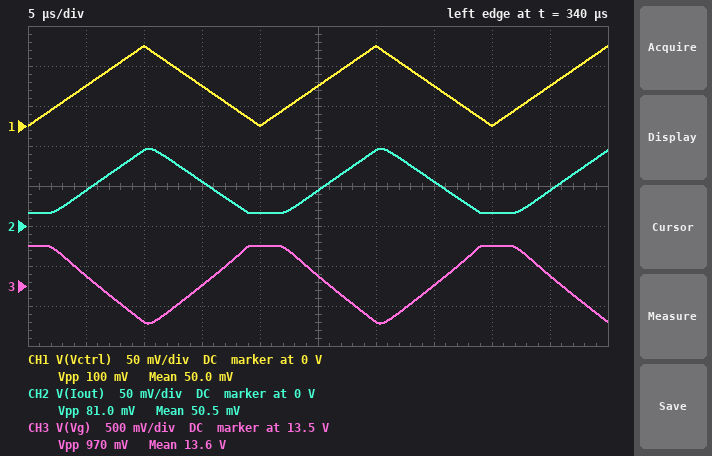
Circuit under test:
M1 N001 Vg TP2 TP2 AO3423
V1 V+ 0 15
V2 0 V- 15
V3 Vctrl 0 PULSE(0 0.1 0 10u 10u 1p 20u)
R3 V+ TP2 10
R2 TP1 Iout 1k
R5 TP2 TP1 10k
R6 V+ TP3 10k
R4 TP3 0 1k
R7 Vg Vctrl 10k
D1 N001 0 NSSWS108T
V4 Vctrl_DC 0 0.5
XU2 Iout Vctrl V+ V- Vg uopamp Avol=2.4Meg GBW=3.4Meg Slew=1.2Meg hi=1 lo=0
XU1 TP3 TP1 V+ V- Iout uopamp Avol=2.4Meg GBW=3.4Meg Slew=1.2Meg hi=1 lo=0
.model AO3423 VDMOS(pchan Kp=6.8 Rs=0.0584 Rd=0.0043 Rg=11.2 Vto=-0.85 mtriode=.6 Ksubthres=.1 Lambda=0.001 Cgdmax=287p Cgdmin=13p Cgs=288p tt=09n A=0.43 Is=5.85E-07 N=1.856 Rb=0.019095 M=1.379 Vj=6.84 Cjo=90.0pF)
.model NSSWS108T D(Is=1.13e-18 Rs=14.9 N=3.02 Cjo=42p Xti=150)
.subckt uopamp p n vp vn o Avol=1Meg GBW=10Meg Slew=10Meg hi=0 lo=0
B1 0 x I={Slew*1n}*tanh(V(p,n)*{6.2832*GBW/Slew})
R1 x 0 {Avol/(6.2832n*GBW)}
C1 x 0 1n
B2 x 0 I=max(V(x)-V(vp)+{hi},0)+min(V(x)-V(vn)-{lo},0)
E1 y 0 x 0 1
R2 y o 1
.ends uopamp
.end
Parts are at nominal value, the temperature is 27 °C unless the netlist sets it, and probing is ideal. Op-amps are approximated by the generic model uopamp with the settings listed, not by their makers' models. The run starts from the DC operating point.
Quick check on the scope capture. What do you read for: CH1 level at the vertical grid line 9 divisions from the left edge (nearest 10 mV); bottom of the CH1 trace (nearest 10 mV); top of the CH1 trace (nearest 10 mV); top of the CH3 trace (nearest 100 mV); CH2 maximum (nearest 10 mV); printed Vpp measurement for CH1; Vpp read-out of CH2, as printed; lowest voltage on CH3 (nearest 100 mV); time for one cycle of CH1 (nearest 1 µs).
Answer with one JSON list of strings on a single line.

["50 mV", "0 V", "100 mV", "14.0 V", "100 mV", "100 mV", "81.0 mV", "13.0 V", "20 µs"]
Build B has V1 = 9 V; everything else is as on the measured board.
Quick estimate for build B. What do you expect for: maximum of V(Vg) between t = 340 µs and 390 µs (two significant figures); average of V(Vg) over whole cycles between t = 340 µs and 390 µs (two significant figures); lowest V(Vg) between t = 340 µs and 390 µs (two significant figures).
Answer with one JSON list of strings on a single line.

["8.0 V", "7.6 V", "7.0 V"]
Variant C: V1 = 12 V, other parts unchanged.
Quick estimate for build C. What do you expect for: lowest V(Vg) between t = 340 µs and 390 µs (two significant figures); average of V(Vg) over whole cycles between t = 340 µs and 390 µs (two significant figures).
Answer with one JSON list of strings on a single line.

["10 V", "11 V"]
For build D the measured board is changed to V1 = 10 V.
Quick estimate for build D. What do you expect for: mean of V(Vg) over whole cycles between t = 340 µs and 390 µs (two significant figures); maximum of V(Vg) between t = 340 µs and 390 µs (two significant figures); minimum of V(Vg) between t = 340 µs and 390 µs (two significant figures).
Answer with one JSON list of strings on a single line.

["8.6 V", "9.0 V", "8.0 V"]
